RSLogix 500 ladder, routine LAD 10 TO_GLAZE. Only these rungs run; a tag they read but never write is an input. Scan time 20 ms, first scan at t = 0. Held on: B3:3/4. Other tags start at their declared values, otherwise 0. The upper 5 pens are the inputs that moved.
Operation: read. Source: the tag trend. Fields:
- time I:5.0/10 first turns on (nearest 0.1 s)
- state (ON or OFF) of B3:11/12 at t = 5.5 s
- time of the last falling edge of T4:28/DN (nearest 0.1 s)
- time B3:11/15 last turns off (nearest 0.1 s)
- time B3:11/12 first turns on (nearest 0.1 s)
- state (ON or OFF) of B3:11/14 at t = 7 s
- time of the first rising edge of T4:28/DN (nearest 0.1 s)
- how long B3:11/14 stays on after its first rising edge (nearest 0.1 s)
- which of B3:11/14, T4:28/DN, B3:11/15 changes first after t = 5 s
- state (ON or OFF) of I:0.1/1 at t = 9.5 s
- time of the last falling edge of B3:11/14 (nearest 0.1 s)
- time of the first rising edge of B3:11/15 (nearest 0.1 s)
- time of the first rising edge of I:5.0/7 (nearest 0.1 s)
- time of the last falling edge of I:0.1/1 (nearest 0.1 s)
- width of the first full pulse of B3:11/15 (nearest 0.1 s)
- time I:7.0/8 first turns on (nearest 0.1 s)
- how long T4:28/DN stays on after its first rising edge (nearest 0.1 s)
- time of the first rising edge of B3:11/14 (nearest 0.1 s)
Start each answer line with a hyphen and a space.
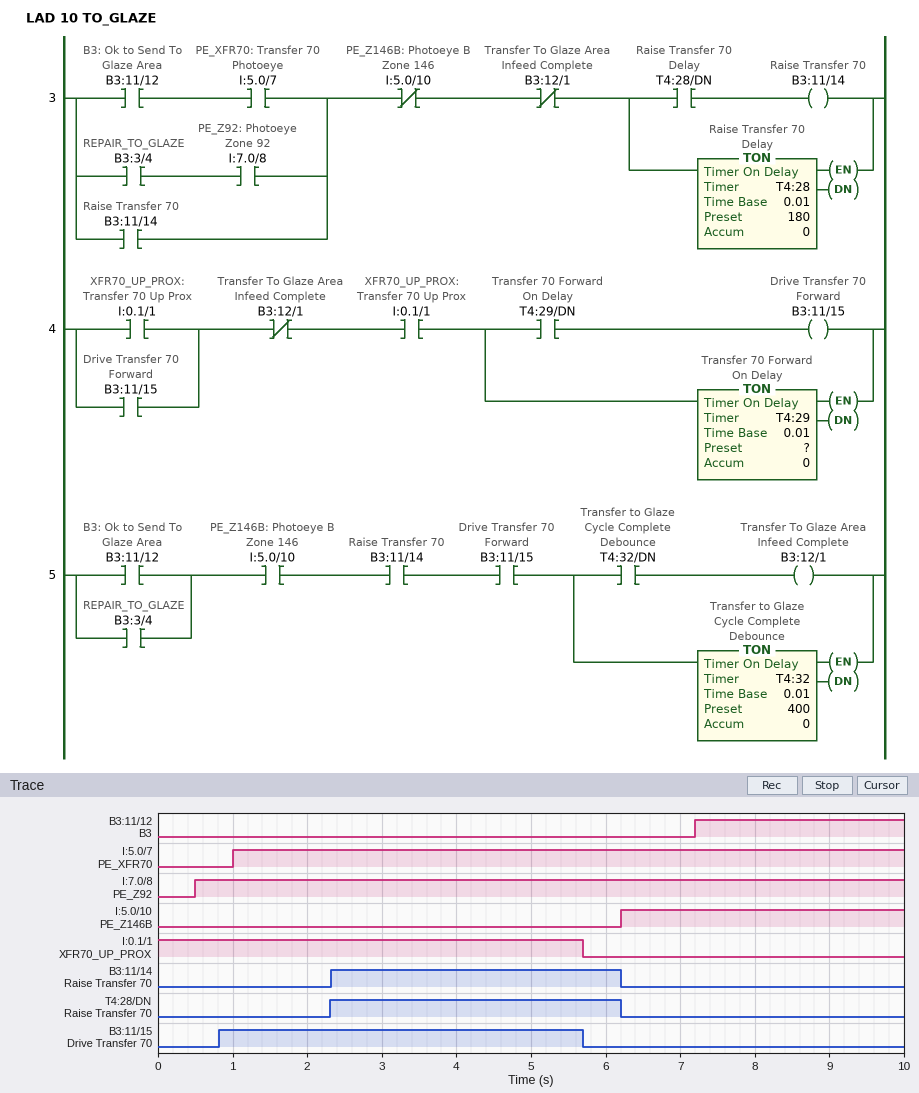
- 6.2 s
- OFF
- 6.2 s
- 5.7 s
- 7.2 s
- OFF
- 2.3 s
- 3.9 s
- B3:11/15
- OFF
- 6.2 s
- 0.8 s
- 1.0 s
- 5.7 s
- 4.9 s
- 0.5 s
- 3.9 s
- 2.3 s
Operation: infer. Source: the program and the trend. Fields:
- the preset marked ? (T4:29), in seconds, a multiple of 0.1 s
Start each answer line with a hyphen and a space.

- 0.8 s
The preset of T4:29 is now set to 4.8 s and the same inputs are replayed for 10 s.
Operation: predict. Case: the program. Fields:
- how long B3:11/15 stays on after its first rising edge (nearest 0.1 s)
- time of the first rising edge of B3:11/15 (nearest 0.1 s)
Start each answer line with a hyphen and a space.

- 0.9 s
- 4.8 s
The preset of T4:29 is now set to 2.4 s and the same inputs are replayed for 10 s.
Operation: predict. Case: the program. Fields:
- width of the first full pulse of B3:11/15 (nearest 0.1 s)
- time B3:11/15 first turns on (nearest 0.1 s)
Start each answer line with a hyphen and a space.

- 3.3 s
- 2.4 s
